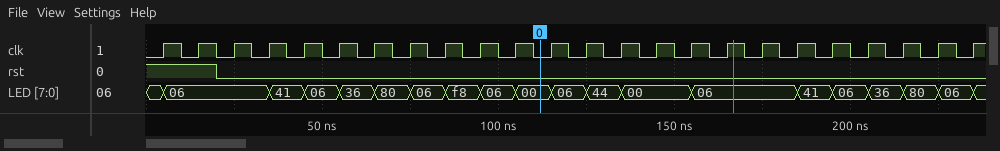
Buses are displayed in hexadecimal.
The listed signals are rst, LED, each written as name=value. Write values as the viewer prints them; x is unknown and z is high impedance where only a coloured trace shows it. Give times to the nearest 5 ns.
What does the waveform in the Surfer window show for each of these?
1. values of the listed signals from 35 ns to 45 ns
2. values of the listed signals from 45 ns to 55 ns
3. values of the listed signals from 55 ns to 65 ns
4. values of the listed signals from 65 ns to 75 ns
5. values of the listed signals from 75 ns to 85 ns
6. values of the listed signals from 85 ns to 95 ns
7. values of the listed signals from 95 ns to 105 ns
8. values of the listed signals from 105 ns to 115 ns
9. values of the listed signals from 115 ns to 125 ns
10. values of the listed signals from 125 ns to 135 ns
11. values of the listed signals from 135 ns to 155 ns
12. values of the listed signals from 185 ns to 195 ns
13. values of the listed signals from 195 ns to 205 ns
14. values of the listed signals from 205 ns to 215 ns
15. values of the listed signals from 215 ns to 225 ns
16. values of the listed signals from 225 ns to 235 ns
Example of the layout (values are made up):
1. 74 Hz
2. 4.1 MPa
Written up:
1. rst=0, LED=41
2. rst=0, LED=06
3. rst=0, LED=36
4. rst=0, LED=80
5. rst=0, LED=06
6. rst=0, LED=f8
7. rst=0, LED=06
8. rst=0, LED=00
9. rst=0, LED=06
10. rst=0, LED=44
11. rst=0, LED=00
12. rst=0, LED=41
13. rst=0, LED=06
14. rst=0, LED=36
15. rst=0, LED=80
16. rst=0, LED=06
